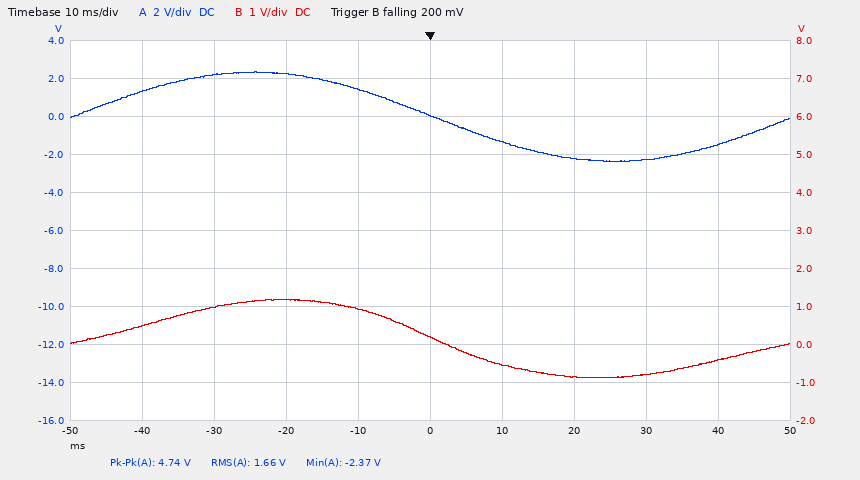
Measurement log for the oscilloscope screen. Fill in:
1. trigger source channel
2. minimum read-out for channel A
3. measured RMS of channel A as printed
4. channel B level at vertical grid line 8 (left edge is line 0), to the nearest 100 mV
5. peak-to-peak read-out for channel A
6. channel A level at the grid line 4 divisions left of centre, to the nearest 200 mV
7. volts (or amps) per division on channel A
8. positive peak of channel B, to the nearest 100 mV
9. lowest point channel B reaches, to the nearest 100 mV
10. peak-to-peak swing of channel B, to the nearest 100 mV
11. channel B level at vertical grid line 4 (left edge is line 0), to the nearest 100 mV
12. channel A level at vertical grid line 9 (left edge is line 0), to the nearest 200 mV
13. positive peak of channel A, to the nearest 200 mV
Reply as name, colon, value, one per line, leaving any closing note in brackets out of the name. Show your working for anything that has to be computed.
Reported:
trigger source channel: channel B
minimum read-out for channel A: -2.37 V
measured RMS of channel A as printed: 1.66 V
channel B level at vertical grid line 8 (left edge is line 0), to the nearest 100 mV: -800 mV
peak-to-peak read-out for channel A: 4.74 V
channel A level at the grid line 4 divisions left of centre, to the nearest 200 mV: 1.4 V
volts (or amps) per division on channel A: 2 V
positive peak of channel B, to the nearest 100 mV: 1.2 V
lowest point channel B reaches, to the nearest 100 mV: -900 mV
peak-to-peak swing of channel B, to the nearest 100 mV: 1.2 V − (-900 mV) = 2.1 V
channel B level at vertical grid line 4 (left edge is line 0), to the nearest 100 mV: 900 mV
channel A level at vertical grid line 9 (left edge is line 0), to the nearest 200 mV: -1.4 V
positive peak of channel A, to the nearest 200 mV: 2.4 V
